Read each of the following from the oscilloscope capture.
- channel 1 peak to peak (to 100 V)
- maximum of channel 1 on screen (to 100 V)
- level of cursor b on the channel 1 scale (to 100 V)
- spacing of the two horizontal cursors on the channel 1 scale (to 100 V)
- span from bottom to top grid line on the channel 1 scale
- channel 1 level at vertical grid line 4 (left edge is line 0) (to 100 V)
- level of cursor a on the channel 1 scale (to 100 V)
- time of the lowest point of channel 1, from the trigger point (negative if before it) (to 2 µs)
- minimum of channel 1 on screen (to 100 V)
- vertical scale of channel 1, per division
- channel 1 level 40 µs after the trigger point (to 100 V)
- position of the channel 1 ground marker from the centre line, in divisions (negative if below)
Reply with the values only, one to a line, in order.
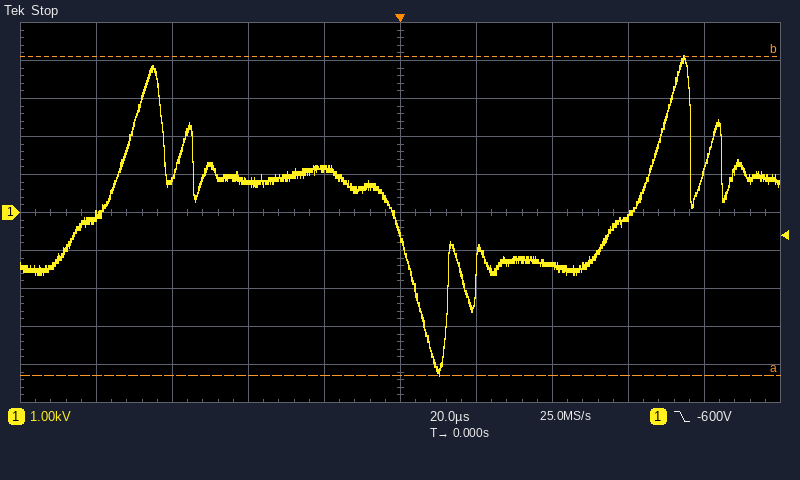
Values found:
8.4 kV
4.1 kV
4.1 kV
8.4 kV
10 kV
1.2 kV
-4.3 kV
+10 µs
-4.3 kV
1 kV
-1.4 kV
0.0 div
